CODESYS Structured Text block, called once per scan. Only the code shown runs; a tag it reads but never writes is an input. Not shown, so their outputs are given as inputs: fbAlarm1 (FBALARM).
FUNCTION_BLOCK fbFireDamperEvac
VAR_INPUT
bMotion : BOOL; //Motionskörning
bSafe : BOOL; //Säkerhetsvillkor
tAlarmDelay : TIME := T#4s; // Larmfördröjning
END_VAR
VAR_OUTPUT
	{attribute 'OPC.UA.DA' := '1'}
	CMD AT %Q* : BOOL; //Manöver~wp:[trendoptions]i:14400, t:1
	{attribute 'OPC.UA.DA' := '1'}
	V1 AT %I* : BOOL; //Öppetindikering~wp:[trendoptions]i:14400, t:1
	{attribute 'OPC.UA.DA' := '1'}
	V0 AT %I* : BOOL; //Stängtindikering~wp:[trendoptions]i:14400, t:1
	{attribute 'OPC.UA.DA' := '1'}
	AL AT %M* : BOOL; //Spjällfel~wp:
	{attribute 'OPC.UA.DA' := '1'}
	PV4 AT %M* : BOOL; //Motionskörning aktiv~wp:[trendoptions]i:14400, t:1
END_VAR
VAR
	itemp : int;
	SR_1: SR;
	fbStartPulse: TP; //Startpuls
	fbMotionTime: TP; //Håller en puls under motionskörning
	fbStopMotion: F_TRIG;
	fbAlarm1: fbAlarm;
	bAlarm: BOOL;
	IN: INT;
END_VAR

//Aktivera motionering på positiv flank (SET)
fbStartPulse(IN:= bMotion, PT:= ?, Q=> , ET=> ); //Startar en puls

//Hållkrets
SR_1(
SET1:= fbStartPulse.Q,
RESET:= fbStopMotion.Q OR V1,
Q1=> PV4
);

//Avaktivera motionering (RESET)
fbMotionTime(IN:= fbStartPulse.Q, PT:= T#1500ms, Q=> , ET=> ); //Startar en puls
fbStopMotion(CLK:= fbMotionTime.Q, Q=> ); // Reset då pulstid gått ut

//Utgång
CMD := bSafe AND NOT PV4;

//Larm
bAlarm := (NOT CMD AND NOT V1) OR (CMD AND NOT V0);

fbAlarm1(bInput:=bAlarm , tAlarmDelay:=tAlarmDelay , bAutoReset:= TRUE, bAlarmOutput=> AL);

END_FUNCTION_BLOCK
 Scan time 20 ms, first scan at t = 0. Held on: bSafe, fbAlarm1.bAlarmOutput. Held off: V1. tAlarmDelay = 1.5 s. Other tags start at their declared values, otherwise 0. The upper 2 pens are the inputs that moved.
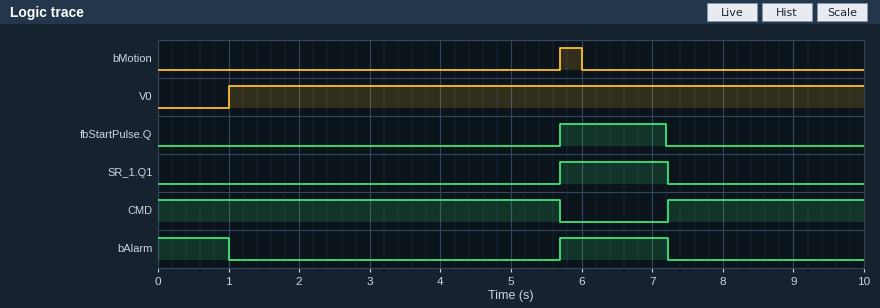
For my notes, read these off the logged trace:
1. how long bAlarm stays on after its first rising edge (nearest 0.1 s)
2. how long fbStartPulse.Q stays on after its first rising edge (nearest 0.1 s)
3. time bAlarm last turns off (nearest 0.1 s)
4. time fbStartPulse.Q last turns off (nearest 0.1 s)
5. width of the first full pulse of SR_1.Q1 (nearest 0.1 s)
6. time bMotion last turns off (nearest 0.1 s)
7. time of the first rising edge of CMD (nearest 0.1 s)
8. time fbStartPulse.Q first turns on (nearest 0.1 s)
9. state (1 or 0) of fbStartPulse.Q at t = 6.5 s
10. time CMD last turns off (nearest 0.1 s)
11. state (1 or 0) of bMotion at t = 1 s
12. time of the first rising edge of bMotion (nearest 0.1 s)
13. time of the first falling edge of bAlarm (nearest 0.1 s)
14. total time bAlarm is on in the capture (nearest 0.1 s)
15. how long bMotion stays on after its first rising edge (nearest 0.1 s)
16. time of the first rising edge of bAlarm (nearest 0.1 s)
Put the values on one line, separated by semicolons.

1.5 s; 1.5 s; 7.2 s; 7.2 s; 1.5 s; 6.0 s; 7.2 s; 5.7 s; 1; 5.7 s; 0; 5.7 s; 1.0 s; 2.5 s; 0.3 s; 5.7 s
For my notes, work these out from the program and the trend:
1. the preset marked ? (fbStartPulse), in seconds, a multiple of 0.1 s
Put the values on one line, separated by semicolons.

1.5 s
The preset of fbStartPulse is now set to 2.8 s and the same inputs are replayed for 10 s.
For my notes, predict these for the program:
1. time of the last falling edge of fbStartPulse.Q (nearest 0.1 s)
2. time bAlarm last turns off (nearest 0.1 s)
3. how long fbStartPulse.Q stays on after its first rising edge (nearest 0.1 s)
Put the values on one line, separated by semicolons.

8.5 s; 1.0 s; 2.8 s
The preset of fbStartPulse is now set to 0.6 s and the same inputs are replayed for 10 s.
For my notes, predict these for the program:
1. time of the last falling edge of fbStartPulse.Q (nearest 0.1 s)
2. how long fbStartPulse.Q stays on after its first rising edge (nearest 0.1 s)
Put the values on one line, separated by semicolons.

6.3 s; 0.6 s
